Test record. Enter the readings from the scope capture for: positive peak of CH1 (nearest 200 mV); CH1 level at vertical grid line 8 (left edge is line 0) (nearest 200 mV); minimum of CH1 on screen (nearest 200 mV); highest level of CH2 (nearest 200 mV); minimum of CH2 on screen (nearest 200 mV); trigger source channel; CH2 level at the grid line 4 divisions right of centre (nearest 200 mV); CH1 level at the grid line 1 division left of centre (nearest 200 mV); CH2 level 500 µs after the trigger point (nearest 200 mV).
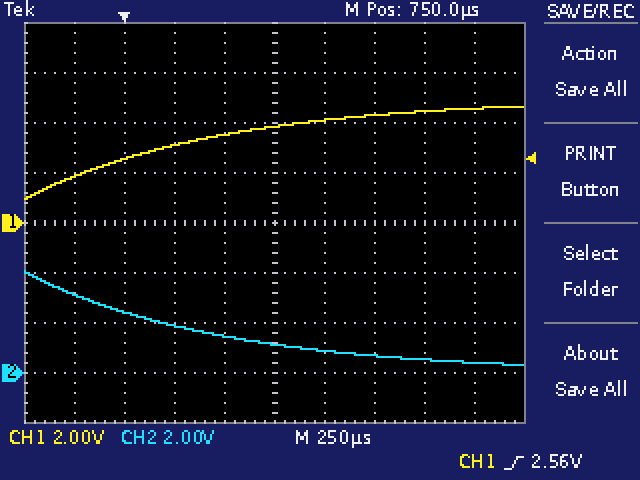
4.6 V
4.4 V
1.0 V
4.0 V
400 mV
CH1
400 mV
3.6 V
1.4 V
